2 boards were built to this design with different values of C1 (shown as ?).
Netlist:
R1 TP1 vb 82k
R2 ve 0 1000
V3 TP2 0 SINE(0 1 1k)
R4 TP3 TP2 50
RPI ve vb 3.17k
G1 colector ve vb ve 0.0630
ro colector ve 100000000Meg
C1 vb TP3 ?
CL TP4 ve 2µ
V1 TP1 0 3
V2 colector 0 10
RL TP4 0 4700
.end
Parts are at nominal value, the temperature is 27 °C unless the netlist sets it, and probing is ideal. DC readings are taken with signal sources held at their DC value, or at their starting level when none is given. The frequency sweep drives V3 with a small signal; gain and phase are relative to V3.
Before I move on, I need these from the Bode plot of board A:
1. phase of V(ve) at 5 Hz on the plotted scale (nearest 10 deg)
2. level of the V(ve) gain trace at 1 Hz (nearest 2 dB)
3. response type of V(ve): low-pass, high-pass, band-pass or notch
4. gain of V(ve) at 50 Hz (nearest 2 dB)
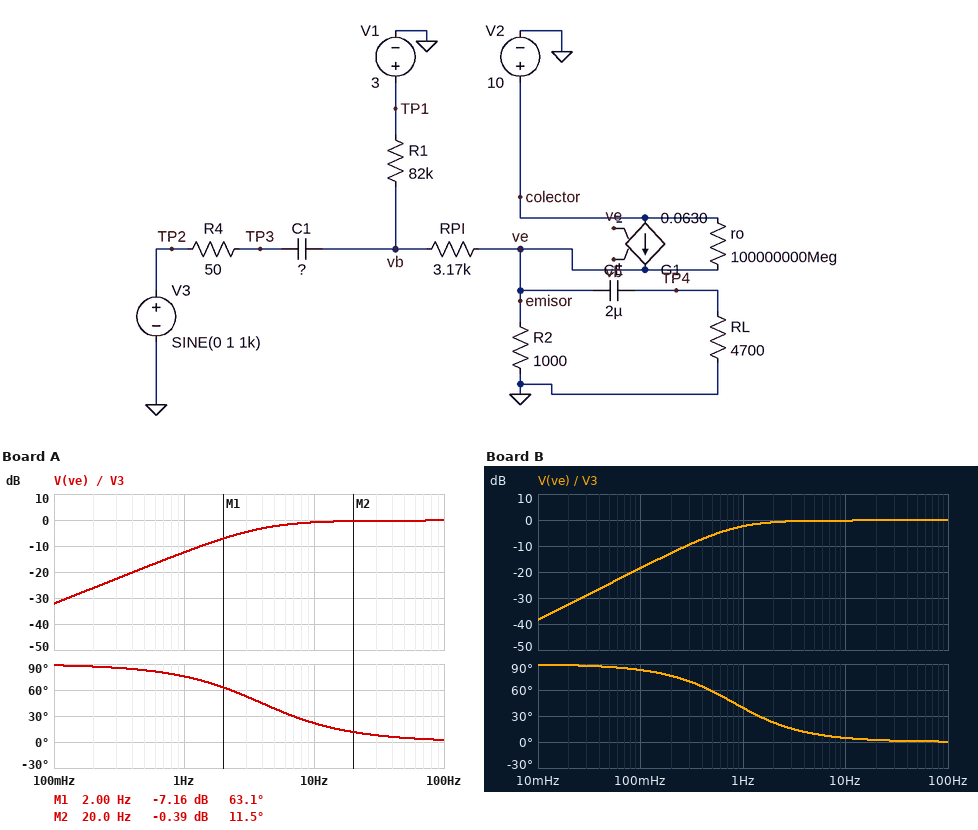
40 deg
-12 dB
high-pass
0 dB
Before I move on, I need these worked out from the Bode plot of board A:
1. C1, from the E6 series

680 nF
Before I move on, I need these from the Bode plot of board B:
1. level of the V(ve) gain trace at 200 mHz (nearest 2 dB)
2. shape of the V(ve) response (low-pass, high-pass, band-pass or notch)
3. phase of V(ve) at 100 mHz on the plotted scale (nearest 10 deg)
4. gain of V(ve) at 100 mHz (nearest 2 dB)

-12 dB
high-pass
80 deg
-18 dB
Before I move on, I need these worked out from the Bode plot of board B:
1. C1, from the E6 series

3.3 µF
